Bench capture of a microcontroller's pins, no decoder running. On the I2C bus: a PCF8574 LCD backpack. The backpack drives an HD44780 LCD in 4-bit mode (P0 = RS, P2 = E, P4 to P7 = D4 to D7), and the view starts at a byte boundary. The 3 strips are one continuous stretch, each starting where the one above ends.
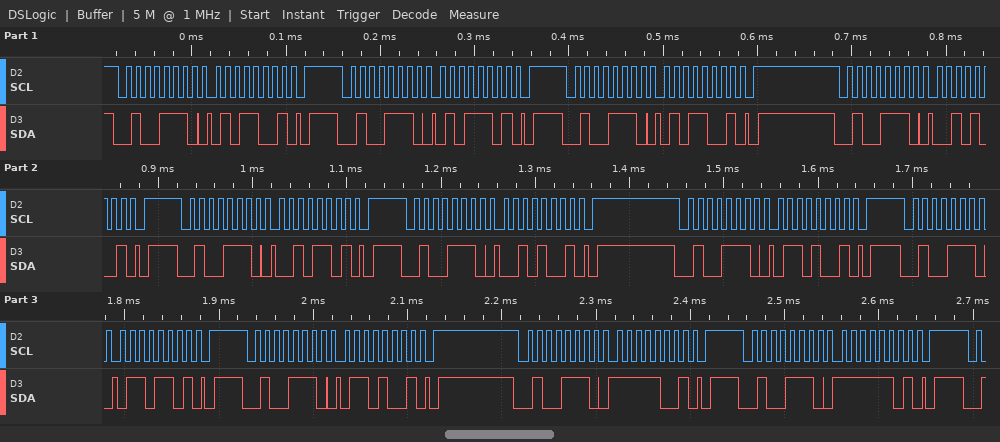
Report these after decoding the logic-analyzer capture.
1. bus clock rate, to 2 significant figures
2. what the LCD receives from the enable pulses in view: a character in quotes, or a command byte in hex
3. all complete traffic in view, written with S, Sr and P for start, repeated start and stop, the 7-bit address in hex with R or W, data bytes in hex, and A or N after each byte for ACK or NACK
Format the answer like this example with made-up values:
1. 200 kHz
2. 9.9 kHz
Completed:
1. 100 kHz
2. 'R'
3. S 27W A 59 A P S 27W A 5D A P S 27W A 59 A P S 27W A 29 A P S 27W A 2D A P S 27W A 29 A P S 27W A 69 A P S 27W A 6D A P S 27W A 69 A P S 27W A F9 A P S 27W A FD A P
